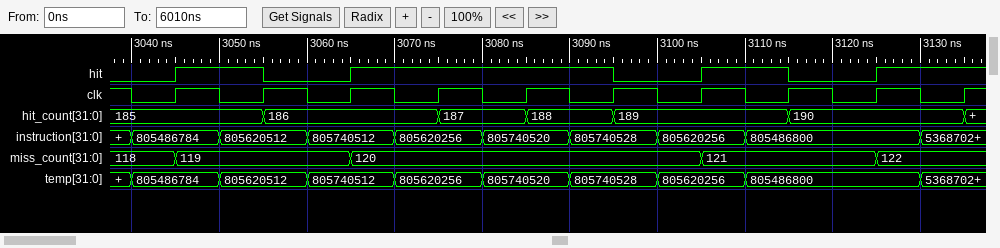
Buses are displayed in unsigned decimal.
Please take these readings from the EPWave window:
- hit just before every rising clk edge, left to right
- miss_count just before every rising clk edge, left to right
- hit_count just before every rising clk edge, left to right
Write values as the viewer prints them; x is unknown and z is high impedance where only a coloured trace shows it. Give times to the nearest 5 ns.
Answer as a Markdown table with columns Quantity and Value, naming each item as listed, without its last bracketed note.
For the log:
| Quantity | Value |
|---|---|
| hit just before every rising clk edge, left to right | 0 1 0 1 1 1 0 1 0 1 |
| miss_count just before every rising clk edge, left to right | 118, 119, 119, 120, 120, 120, 120, 121, 121, 122 |
| hit_count just before every rising clk edge, left to right | 185, 185, 186, 186, 187, 188, 189, 189, 190, 190 |
